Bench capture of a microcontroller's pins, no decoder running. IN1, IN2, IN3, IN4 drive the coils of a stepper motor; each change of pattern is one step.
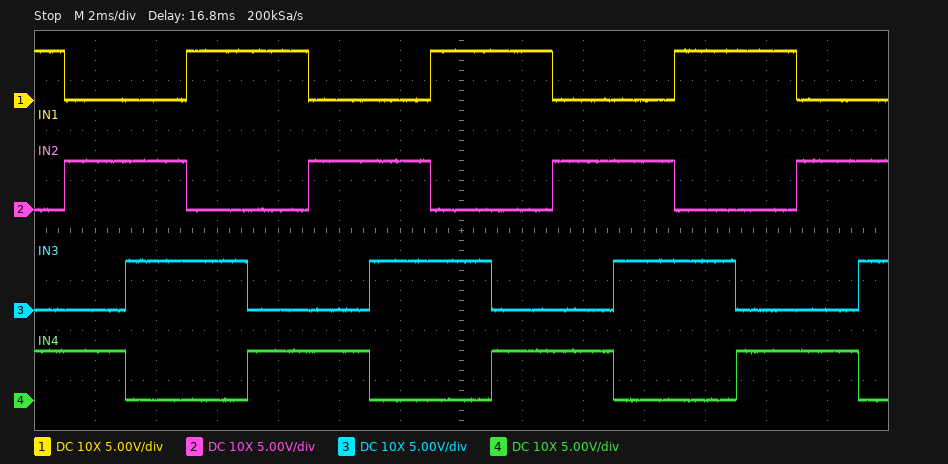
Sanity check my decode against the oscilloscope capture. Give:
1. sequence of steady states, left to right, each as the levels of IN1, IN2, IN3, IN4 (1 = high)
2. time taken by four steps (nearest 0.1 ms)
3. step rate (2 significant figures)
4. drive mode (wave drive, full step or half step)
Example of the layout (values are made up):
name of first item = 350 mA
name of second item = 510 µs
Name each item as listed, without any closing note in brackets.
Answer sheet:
sequence of steady states, left to right, each as the levels of IN1, IN2, IN3, IN4 = 1001 0101 0110 1010 1001 0101 0110 1010 1001 0101 0110 1010 1001 0101 0110
time taken by four steps = 8.0 ms
step rate = 500 steps/s
drive mode = full step
